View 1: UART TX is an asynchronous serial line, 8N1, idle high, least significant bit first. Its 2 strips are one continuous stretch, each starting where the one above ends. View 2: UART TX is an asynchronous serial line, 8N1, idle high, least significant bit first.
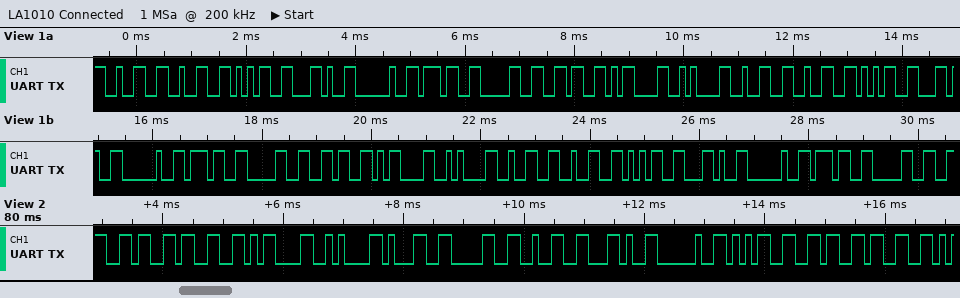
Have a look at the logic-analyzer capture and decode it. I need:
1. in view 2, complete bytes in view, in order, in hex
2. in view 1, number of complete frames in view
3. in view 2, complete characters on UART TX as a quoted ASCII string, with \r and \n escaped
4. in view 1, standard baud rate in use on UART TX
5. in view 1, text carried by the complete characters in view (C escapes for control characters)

36 33 0D 0A 31 30 32 2C 20 35 36 33
27
"63\r\n102, 563"
9600 baud
"225, 706\r\n225, 706\r\n225, 70"
